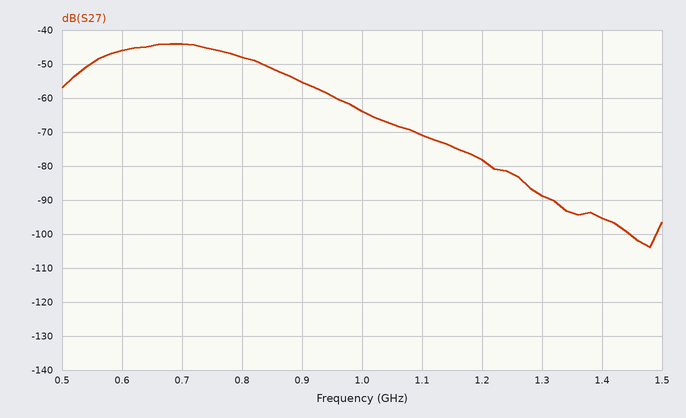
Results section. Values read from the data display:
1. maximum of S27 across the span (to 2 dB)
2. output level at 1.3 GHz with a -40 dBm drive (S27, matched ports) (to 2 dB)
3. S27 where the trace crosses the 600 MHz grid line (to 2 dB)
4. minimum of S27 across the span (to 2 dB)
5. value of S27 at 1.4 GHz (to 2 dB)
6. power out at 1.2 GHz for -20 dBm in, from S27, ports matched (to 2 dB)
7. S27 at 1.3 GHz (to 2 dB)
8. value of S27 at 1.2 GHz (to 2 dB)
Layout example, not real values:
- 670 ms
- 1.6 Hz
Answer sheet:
- -44 dB
- -128 dBm
- -46 dB
- -104 dB
- -96 dB
- -98 dBm
- -88 dB
- -78 dB
